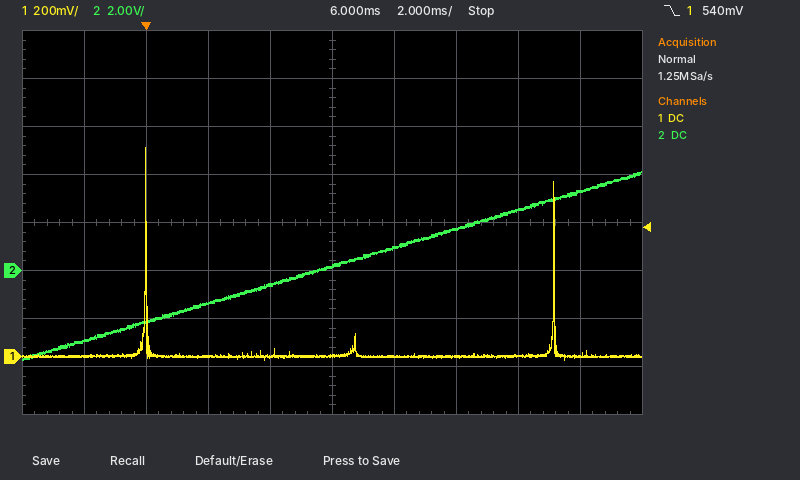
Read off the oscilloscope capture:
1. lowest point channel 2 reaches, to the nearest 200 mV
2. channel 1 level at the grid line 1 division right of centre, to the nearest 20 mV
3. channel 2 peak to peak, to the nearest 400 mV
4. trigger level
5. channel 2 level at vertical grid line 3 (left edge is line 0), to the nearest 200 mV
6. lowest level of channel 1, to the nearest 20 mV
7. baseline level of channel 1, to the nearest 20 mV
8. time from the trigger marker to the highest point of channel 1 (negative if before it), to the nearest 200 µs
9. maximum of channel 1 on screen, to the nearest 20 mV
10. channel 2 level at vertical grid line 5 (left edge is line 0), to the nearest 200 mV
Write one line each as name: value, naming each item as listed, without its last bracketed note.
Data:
lowest point channel 2 reaches, to the nearest 200 mV: -3.8 V
channel 1 level at the grid line 1 division right of centre, to the nearest 20 mV: 0 mV
channel 2 peak to peak, to the nearest 400 mV: 8.0 V
trigger level: 540 mV
channel 2 level at vertical grid line 3 (left edge is line 0), to the nearest 200 mV: -1.4 V
lowest level of channel 1, to the nearest 20 mV: -20 mV
baseline level of channel 1, to the nearest 20 mV: 0 mV
time from the trigger marker to the highest point of channel 1 (negative if before it), to the nearest 200 µs: 0.0 ms
maximum of channel 1 on screen, to the nearest 20 mV: 880 mV
channel 2 level at vertical grid line 5 (left edge is line 0), to the nearest 200 mV: 200 mV
